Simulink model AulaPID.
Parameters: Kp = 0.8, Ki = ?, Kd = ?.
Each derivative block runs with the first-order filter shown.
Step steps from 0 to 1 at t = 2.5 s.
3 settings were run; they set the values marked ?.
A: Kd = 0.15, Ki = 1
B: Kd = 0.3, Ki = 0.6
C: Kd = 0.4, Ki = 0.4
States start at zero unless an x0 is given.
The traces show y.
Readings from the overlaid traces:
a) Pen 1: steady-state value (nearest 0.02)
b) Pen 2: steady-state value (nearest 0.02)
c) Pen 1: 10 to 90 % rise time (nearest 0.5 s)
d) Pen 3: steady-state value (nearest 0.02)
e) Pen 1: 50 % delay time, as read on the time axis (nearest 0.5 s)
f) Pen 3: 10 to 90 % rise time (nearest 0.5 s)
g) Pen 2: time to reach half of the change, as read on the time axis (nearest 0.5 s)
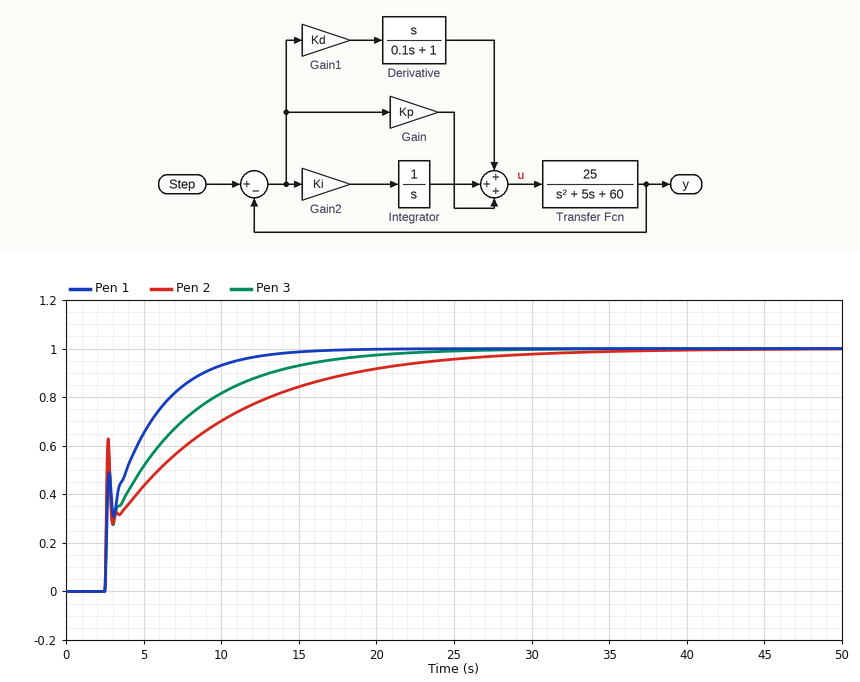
1.00
1.00
6.5 s
1.00
4.0 s
10.5 s
2.5 s
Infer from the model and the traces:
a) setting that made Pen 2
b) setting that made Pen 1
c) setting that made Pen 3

C
A
B
